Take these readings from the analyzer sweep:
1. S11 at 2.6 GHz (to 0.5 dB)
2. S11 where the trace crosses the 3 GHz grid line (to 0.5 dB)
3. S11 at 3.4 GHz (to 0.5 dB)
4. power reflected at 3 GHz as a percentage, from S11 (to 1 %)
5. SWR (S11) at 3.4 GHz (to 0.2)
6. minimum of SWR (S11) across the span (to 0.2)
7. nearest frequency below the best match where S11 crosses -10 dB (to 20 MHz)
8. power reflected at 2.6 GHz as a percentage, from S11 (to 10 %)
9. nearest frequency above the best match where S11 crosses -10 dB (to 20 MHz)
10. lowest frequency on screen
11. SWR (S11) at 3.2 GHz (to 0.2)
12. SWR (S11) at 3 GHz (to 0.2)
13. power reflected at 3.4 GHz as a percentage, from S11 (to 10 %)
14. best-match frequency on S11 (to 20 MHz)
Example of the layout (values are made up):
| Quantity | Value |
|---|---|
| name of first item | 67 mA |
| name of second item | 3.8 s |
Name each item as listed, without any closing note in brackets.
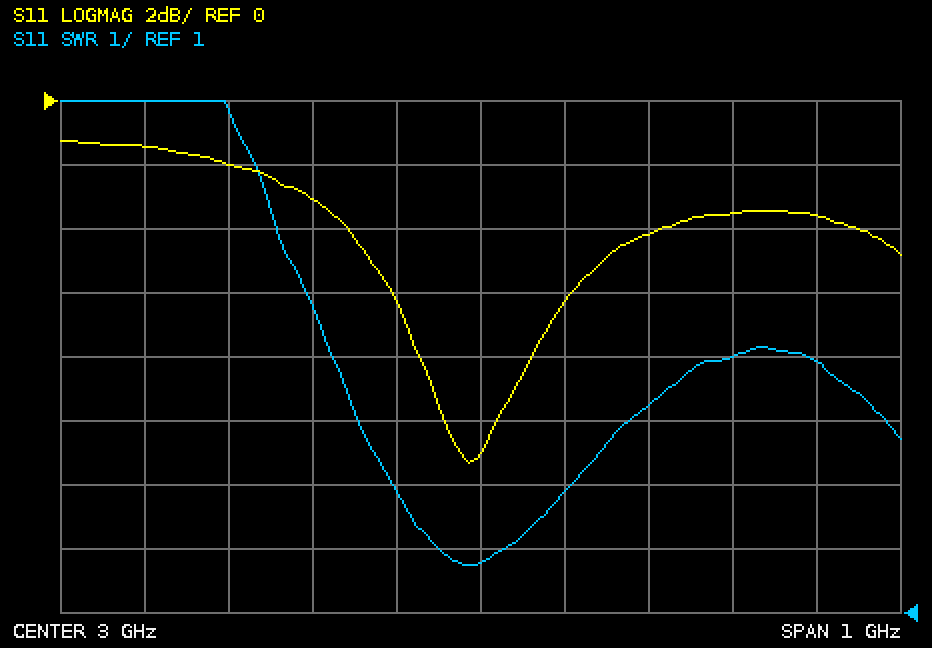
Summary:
| Quantity | Value |
|---|---|
| S11 at 2.6 GHz | -1.5 dB |
| S11 where the trace crosses the 3 GHz grid line | -11.0 dB |
| S11 at 3.4 GHz | -3.5 dB |
| power reflected at 3 GHz as a percentage, from S11 | 8 % |
| SWR (S11) at 3.4 GHz | 5.0 |
| minimum of SWR (S11) across the span | 1.8 |
| nearest frequency below the best match where S11 crosses -10 dB | 2.96 GHz |
| power reflected at 2.6 GHz as a percentage, from S11 | 70 % |
| nearest frequency above the best match where S11 crosses -10 dB | 3.02 GHz |
| lowest frequency on screen | 2.5 GHz |
| SWR (S11) at 3.2 GHz | 4.2 |
| SWR (S11) at 3 GHz | 1.8 |
| power reflected at 3.4 GHz as a percentage, from S11 | 40 % |
| best-match frequency on S11 | 2.98 GHz |
